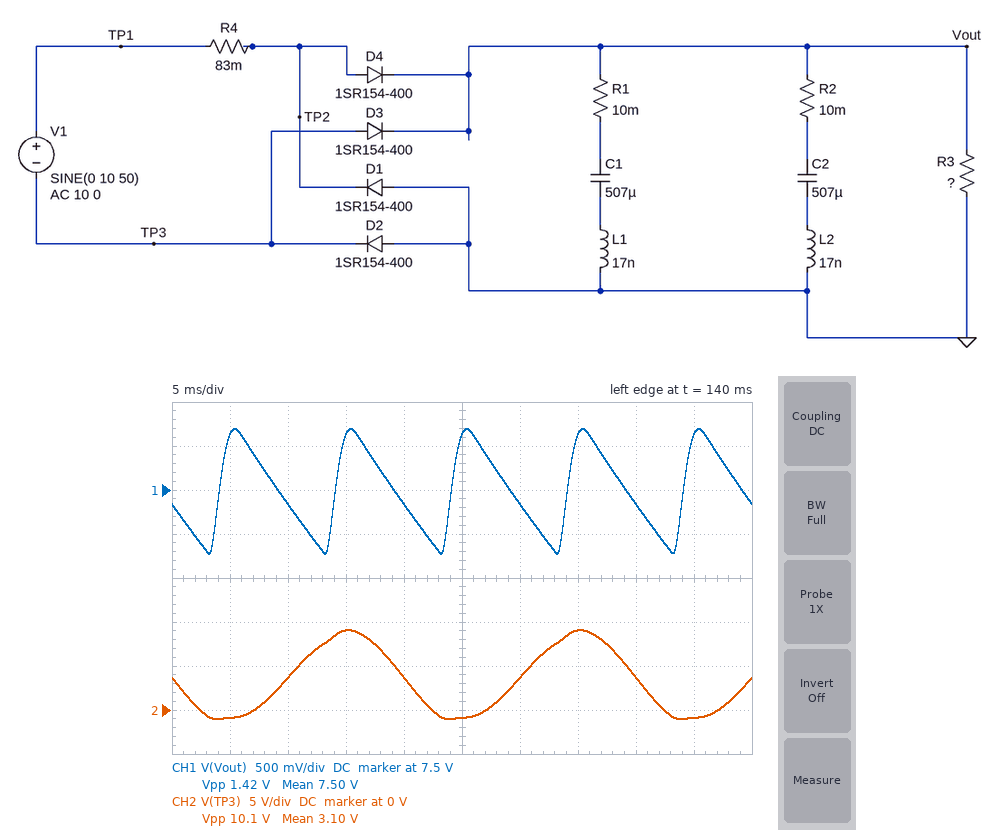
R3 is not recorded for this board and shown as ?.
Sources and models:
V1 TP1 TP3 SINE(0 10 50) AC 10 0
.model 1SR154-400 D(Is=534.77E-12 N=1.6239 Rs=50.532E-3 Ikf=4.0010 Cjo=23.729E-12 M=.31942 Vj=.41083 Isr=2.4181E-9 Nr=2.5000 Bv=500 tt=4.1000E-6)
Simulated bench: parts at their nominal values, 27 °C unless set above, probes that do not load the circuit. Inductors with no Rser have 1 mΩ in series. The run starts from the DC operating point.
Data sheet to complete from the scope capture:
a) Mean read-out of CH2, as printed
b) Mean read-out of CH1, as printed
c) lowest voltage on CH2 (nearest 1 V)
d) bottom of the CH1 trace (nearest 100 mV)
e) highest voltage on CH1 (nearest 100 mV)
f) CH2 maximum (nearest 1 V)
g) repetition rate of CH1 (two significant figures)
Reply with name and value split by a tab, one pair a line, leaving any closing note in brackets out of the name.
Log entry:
Mean read-out of CH2, as printed	3.10 V
Mean read-out of CH1, as printed	7.50 V
lowest voltage on CH2	-1 V
bottom of the CH1 trace	6.8 V
highest voltage on CH1	8.2 V
CH2 maximum	9 V
repetition rate of CH1	100 Hz
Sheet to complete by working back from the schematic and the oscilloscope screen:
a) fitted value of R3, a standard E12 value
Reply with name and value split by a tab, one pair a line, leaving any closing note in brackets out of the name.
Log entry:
fitted value of R3, a standard E12 value	39 Ω
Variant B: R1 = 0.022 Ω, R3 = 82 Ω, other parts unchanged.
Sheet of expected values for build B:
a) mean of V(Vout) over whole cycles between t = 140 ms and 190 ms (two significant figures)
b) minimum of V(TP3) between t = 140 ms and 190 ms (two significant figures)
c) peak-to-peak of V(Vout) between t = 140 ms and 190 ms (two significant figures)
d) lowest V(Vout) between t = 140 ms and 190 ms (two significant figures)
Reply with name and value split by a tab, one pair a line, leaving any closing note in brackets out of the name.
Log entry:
mean of V(Vout) over whole cycles between t = 140 ms and 190 ms	7.9 V
minimum of V(TP3) between t = 140 ms and 190 ms	-950 mV
peak-to-peak of V(Vout) between t = 140 ms and 190 ms	750 mV
lowest V(Vout) between t = 140 ms and 190 ms	7.5 V
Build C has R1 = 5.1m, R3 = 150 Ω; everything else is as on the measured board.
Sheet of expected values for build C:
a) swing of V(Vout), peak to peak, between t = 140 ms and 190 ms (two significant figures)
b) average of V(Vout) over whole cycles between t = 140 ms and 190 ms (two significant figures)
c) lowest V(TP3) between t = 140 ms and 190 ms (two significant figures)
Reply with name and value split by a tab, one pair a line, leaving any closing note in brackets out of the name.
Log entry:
swing of V(Vout), peak to peak, between t = 140 ms and 190 ms	430 mV
average of V(Vout) over whole cycles between t = 140 ms and 190 ms	8.1 V
lowest V(TP3) between t = 140 ms and 190 ms	-910 mV
